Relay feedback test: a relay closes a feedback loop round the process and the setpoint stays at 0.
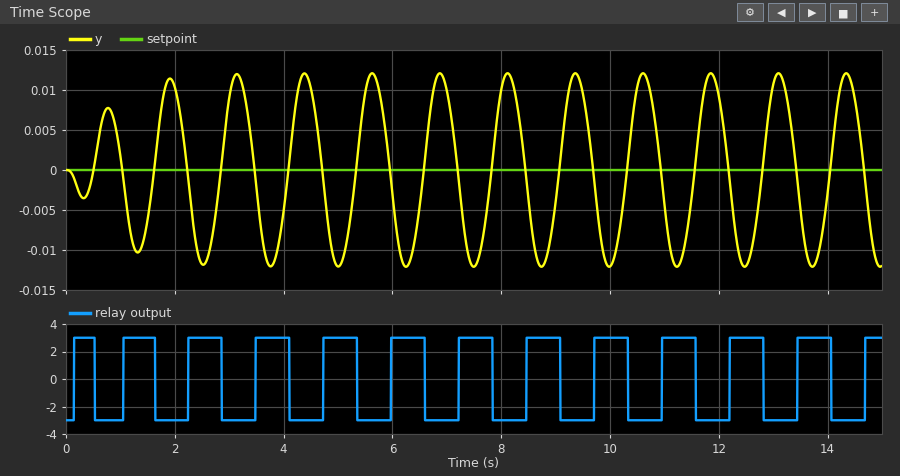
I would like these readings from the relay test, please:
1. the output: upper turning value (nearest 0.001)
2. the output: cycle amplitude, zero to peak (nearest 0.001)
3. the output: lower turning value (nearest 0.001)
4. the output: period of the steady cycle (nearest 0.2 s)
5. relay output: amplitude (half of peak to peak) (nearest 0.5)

0.012
0.012
-0.012
1.2 s
3.0
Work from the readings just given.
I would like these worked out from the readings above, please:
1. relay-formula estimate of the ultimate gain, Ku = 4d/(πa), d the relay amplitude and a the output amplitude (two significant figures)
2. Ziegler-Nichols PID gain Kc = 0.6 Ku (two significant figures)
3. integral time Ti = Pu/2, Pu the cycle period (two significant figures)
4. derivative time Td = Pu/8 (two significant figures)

320
190
0.60 s
0.15 s
